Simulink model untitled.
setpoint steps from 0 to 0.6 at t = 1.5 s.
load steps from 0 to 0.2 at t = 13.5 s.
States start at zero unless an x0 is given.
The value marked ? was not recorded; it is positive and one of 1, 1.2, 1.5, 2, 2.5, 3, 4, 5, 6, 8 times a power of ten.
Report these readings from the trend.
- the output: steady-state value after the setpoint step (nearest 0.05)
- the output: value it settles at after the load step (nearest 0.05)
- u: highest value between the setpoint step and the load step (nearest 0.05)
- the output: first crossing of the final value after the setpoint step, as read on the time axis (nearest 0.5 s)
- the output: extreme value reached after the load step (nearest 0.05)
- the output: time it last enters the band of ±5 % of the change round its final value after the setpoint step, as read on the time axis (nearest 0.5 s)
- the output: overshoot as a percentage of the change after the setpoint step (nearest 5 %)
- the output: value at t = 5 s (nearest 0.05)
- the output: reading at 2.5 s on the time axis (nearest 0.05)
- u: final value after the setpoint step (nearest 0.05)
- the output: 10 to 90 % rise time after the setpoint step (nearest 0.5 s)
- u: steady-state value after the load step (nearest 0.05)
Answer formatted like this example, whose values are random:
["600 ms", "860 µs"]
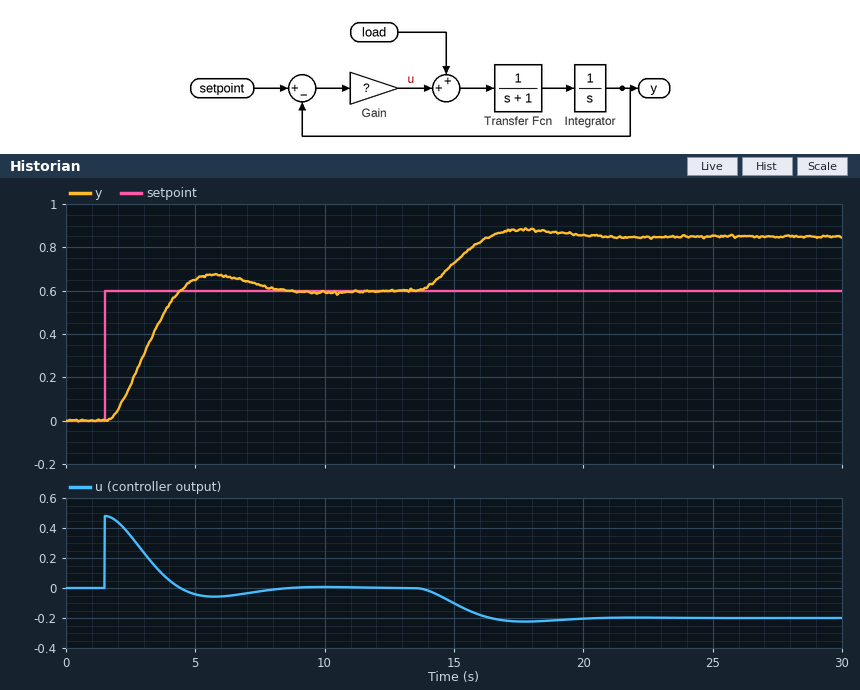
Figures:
["0.60", "0.85", "0.50", "4.5 s", "0.90", "7.5 s", "10 %", "0.65", "0.15", "0.00", "2.0 s", "-0.20"]
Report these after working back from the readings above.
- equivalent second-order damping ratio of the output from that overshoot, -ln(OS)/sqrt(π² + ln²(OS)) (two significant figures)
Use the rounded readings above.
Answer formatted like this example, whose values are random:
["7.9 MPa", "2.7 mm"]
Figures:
["0.59"]
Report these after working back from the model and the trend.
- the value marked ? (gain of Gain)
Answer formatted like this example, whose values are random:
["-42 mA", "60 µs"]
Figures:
["0.8"]
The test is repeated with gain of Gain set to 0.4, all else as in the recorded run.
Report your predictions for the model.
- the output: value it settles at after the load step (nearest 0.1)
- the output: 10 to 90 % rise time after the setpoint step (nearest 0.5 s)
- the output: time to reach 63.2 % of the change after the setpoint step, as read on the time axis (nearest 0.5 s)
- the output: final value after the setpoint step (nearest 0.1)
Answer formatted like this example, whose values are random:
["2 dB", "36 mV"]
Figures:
["1.1", "4.0 s", "4.5 s", "0.6"]
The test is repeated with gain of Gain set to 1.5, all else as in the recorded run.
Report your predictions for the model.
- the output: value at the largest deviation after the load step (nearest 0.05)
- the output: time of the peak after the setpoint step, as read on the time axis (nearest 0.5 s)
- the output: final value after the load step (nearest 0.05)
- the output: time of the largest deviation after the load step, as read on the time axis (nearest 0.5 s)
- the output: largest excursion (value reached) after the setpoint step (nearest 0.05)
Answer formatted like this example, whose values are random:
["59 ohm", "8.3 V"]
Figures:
["0.75", "4.5 s", "0.75", "16.5 s", "0.75"]
